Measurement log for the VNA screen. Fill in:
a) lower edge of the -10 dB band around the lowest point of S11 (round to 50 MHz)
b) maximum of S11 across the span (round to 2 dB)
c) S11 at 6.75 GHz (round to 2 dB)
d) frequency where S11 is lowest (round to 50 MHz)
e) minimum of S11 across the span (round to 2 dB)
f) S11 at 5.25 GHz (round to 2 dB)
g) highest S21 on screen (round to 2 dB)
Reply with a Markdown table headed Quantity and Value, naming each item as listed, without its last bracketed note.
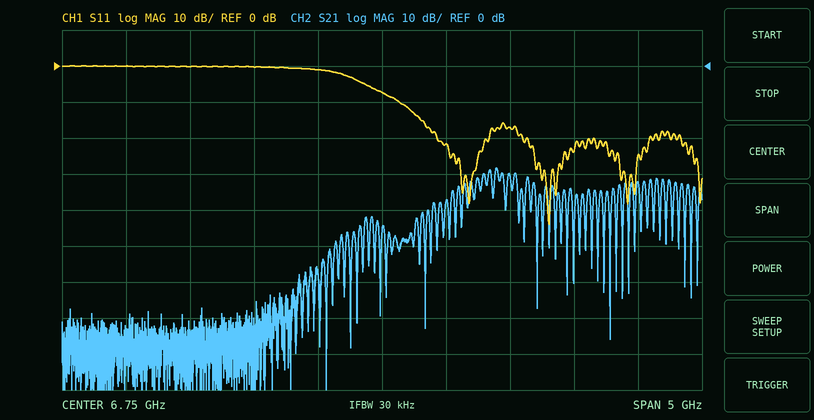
| Quantity | Value |
|---|---|
| lower edge of the -10 dB band around the lowest point of S11 | 6.90 GHz |
| maximum of S11 across the span | 0 dB |
| S11 at 6.75 GHz | -8 dB |
| frequency where S11 is lowest | 8.05 GHz |
| minimum of S11 across the span | -44 dB |
| S11 at 5.25 GHz | 0 dB |
| highest S21 on screen | -28 dB |
